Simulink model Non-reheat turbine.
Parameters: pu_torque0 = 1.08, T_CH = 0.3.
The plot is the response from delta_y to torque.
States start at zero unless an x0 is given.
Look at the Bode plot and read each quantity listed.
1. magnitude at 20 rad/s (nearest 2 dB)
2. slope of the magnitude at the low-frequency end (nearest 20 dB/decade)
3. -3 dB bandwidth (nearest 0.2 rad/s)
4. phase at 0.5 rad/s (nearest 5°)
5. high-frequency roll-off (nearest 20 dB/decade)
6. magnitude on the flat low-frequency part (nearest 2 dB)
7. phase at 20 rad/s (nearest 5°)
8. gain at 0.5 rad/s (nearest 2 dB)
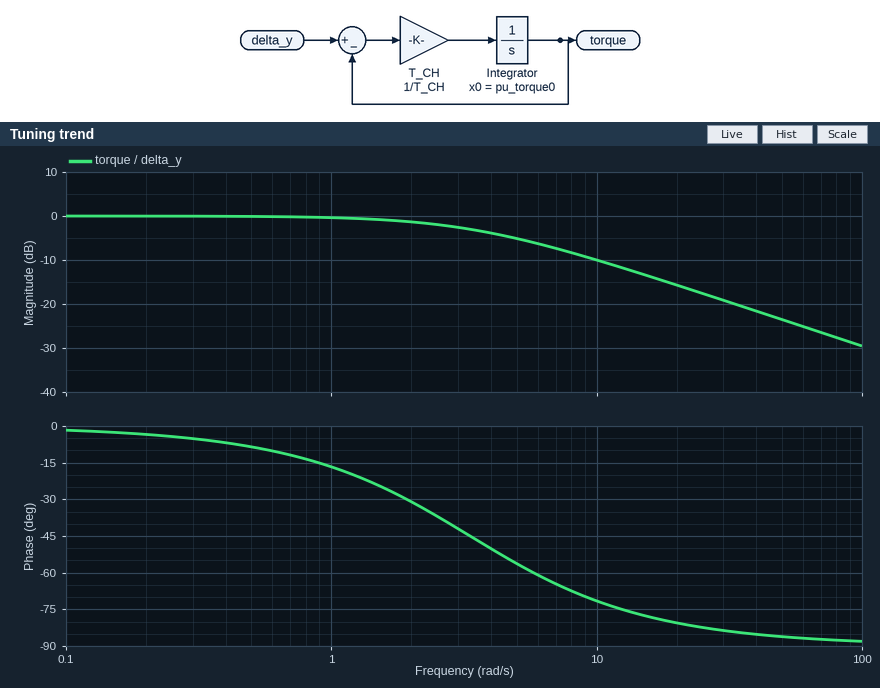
-16 dB
0 dB/decade
3.4 rad/s
-10°
-20 dB/decade
0 dB
-80°
0 dB
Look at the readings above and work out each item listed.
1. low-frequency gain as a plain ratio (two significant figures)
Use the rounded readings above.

1.0
